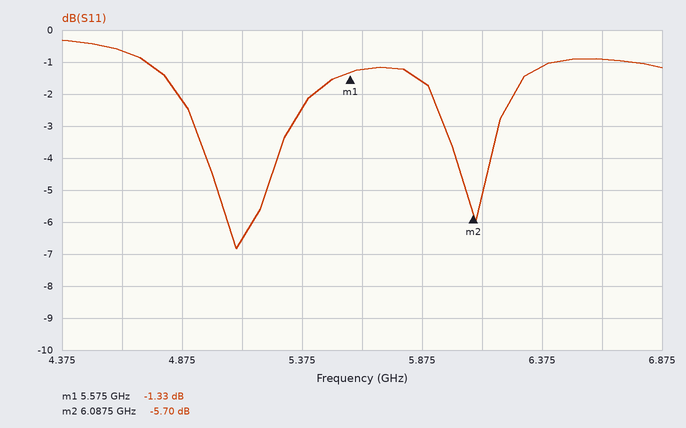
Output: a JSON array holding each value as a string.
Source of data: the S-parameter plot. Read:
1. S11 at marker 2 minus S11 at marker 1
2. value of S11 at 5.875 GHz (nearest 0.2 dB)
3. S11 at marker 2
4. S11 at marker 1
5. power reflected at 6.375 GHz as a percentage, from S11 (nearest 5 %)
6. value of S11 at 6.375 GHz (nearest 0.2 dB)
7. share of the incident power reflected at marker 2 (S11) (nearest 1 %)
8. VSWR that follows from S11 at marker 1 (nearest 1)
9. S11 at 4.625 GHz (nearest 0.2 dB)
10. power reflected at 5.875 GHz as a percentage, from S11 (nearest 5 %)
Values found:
["-4.37 dB", "-1.6 dB", "-5.70 dB", "-1.33 dB", "75 %", "-1.2 dB", "27 %", "13", "-0.6 dB", "70 %"]
